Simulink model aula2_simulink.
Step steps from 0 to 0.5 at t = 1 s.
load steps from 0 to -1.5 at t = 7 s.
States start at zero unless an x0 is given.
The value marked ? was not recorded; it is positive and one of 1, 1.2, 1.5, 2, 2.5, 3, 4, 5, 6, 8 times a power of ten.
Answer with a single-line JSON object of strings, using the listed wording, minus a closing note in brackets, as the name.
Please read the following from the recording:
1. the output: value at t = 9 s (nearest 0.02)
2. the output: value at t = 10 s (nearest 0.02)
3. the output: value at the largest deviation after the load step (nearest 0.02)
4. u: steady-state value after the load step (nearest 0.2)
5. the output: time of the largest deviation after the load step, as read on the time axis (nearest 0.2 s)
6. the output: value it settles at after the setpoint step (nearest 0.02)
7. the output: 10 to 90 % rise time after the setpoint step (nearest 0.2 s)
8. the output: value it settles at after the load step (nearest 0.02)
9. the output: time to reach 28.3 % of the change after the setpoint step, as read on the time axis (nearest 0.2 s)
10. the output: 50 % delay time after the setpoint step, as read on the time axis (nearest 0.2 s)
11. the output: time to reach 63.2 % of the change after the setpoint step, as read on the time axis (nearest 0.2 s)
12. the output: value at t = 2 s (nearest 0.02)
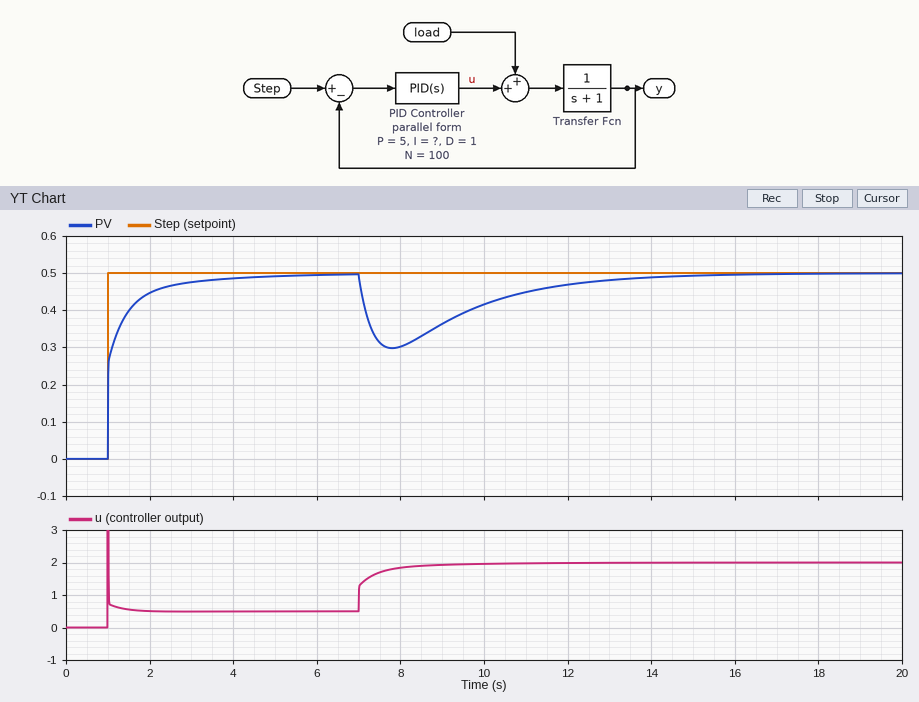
{"the output: value at t = 9 s": "0.36", "the output: value at t = 10 s": "0.42", "the output: value at the largest deviation after the load step": "0.30", "u: steady-state value after the load step": "2.0", "the output: time of the largest deviation after the load step, as read on the time axis": "7.8 s", "the output: value it settles at after the setpoint step": "0.50", "the output: 10 to 90 % rise time after the setpoint step": "1.0 s", "the output: value it settles at after the load step": "0.50", "the output: time to reach 28.3 % of the change after the setpoint step, as read on the time axis": "1.0 s", "the output: 50 % delay time after the setpoint step, as read on the time axis": "1.0 s", "the output: time to reach 63.2 % of the change after the setpoint step, as read on the time axis": "1.2 s", "the output: value at t = 2 s": "0.44"}
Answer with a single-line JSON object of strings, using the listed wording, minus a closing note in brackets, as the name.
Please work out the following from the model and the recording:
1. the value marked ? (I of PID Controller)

{"the value marked ?": "2.5"}
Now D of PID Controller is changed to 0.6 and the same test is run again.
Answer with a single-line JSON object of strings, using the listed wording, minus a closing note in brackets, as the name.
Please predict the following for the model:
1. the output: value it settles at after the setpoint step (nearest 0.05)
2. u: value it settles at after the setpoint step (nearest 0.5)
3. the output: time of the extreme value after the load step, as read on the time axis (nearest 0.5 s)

{"the output: value it settles at after the setpoint step": "0.50", "u: value it settles at after the setpoint step": "0.5", "the output: time of the extreme value after the load step, as read on the time axis": "7.5 s"}
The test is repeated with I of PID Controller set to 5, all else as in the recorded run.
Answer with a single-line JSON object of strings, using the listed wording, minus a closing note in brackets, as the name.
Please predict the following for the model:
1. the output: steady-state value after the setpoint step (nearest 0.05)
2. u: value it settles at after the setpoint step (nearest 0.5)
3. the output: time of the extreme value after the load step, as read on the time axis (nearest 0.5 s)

{"the output: steady-state value after the setpoint step": "0.50", "u: value it settles at after the setpoint step": "0.5", "the output: time of the extreme value after the load step, as read on the time axis": "7.5 s"}
